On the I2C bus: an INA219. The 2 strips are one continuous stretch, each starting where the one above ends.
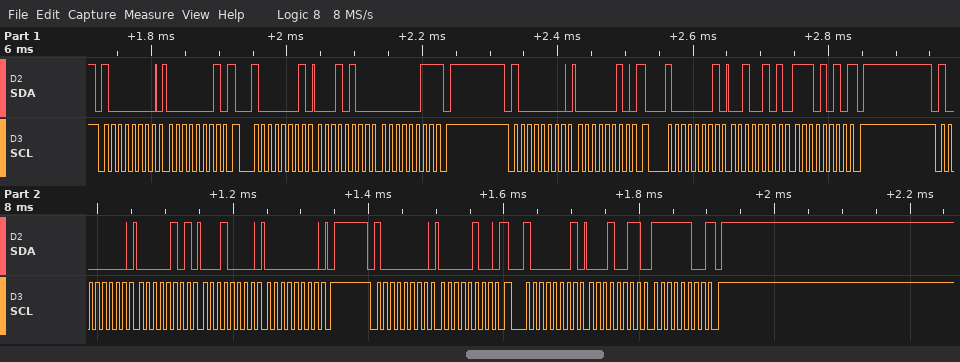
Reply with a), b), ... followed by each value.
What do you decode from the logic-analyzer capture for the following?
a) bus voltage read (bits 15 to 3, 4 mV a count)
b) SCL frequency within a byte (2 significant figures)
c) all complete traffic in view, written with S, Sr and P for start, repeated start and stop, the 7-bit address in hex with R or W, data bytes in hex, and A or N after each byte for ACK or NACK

a) 4.852 V
b) 100 kHz
c) S 40W A 01 A Sr 40R A 14 A 03 N P S 40W A 02 A Sr 40R A 25 A EA N P S 40W A 05 A 10 A 00 A P S 40W A 04 A Sr 40R A 13 A FC N P
